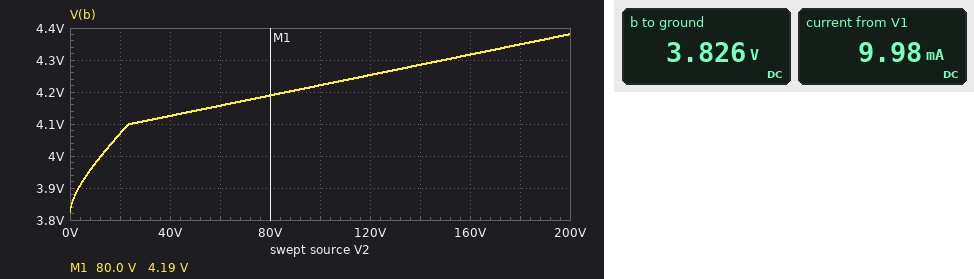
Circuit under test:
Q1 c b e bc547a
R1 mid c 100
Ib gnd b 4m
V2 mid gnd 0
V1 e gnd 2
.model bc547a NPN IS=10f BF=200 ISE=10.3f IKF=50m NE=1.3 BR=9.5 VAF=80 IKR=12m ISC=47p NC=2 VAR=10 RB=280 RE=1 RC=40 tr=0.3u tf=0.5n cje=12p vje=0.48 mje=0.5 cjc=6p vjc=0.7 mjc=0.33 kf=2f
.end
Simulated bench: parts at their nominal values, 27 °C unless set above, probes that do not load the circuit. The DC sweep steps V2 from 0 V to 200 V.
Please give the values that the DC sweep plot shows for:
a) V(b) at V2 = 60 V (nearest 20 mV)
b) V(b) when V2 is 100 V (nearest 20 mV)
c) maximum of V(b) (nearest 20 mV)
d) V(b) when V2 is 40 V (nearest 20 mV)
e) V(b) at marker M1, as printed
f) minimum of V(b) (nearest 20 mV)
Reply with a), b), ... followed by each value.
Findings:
a) 4.16 V
b) 4.22 V
c) 4.38 V
d) 4.12 V
e) 4.19 V
f) 3.82 V
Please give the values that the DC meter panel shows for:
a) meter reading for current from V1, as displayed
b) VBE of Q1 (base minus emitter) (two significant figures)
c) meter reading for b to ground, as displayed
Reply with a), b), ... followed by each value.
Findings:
a) 9.98 mA
b) 1.8 V
c) 3.826 V
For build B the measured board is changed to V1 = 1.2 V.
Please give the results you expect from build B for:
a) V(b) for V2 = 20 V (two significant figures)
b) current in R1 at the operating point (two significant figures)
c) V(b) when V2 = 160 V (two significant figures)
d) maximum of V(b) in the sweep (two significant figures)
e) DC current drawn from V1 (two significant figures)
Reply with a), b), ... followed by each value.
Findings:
a) 3.3 V
b) 8.5 mA
c) 3.5 V
d) 3.6 V
e) 4.5 mA
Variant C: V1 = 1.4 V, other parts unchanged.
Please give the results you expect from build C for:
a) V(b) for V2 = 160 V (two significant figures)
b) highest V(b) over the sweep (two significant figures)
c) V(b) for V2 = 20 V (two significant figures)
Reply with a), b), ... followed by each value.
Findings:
a) 3.7 V
b) 3.8 V
c) 3.5 V
